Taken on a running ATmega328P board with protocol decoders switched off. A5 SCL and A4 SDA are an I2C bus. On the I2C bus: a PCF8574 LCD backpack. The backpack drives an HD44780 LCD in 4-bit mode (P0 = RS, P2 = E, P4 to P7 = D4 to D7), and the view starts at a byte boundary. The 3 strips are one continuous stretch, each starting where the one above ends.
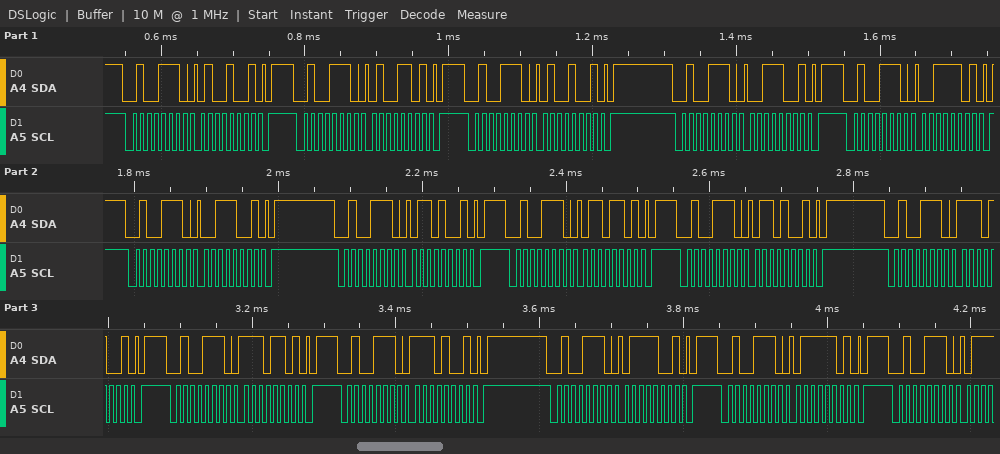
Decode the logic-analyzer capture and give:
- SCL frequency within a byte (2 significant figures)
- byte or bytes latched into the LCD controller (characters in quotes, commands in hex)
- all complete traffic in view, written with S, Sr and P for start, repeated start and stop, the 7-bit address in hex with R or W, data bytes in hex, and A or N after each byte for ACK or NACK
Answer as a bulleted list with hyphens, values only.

- 100 kHz
- 'C' 'n'
- S 27W A 49 A P S 27W A 4D A P S 27W A 49 A P S 27W A 39 A P S 27W A 3D A P S 27W A 39 A P S 27W A 69 A P S 27W A 6D A P S 27W A 69 A P S 27W A E9 A P S 27W A ED A P S 27W A E9 A P S 27W A 79 A P S 27W A 7D A P S 27W A
